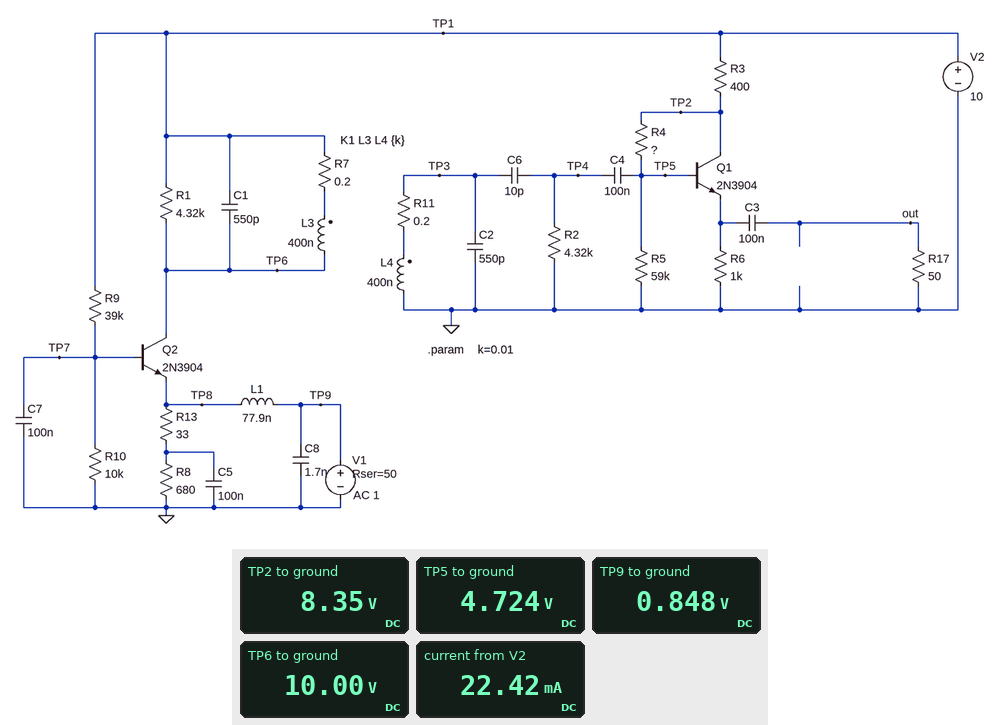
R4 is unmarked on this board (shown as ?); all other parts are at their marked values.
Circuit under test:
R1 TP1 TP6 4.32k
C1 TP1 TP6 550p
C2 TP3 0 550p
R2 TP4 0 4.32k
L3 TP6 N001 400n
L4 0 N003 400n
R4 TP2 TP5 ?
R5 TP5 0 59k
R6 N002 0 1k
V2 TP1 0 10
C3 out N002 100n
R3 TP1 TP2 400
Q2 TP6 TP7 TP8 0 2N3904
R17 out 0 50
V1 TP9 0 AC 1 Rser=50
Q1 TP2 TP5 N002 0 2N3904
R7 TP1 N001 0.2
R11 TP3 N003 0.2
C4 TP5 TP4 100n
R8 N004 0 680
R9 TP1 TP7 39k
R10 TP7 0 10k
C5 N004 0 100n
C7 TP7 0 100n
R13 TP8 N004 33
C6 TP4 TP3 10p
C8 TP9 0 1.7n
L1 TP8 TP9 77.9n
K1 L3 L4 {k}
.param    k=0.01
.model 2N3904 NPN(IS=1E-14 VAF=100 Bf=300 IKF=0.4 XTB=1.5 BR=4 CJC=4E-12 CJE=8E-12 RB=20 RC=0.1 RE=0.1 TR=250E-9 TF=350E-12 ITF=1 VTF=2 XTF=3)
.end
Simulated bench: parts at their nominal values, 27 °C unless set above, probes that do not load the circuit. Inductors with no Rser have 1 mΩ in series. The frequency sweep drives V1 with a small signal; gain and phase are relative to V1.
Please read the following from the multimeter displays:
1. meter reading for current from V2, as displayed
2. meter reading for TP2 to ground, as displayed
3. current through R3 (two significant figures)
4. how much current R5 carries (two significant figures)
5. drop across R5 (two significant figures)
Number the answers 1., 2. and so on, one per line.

1. 22.42 mA
2. 8.35 V
3. 4.1 mA
4. 80 µA
5. 4.7 V
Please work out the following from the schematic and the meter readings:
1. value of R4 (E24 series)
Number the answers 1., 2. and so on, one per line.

1. 39 kΩ
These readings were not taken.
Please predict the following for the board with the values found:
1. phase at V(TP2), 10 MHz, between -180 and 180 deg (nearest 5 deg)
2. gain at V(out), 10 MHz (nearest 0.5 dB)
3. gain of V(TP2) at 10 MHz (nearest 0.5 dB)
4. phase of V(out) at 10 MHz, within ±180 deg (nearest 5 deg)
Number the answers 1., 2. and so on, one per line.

1. 60 deg
2. -17.0 dB
3. 1.5 dB
4. -115 deg
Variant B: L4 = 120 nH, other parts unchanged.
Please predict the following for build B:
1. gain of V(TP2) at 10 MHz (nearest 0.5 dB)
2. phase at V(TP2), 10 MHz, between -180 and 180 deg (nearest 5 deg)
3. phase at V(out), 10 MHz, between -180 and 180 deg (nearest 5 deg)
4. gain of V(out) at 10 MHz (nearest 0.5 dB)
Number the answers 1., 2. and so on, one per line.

1. -19.5 dB
2. 65 deg
3. -110 deg
4. -38.0 dB
